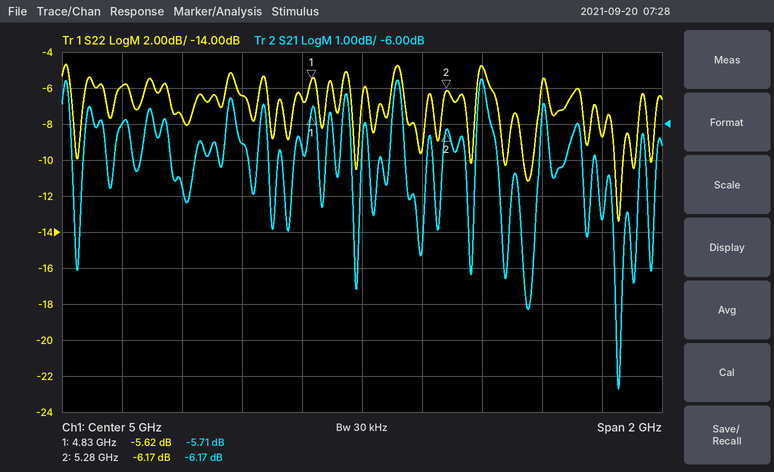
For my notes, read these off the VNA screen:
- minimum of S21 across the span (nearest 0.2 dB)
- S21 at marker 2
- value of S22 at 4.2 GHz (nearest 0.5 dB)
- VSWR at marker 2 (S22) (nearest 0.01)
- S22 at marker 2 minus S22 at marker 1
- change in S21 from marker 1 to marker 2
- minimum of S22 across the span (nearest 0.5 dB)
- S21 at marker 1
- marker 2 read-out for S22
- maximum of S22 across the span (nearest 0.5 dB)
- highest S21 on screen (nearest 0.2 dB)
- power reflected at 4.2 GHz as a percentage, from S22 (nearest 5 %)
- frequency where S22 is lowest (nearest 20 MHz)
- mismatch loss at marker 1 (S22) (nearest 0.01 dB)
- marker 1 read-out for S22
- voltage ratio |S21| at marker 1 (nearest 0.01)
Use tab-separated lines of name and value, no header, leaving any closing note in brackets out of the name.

minimum of S21 across the span	-13.4 dB
S21 at marker 2	-6.17 dB
value of S22 at 4.2 GHz	-6.0 dB
VSWR at marker 2 (S22)	2.93
S22 at marker 2 minus S22 at marker 1	-0.55 dB
change in S21 from marker 1 to marker 2	-0.46 dB
minimum of S22 across the span	-13.5 dB
S21 at marker 1	-5.71 dB
marker 2 read-out for S22	-6.17 dB
maximum of S22 across the span	-4.5 dB
highest S21 on screen	-4.8 dB
power reflected at 4.2 GHz as a percentage, from S22	25 %
frequency where S22 is lowest	5.86 GHz
mismatch loss at marker 1 (S22)	1.39 dB
marker 1 read-out for S22	-5.62 dB
voltage ratio |S21| at marker 1	0.52
